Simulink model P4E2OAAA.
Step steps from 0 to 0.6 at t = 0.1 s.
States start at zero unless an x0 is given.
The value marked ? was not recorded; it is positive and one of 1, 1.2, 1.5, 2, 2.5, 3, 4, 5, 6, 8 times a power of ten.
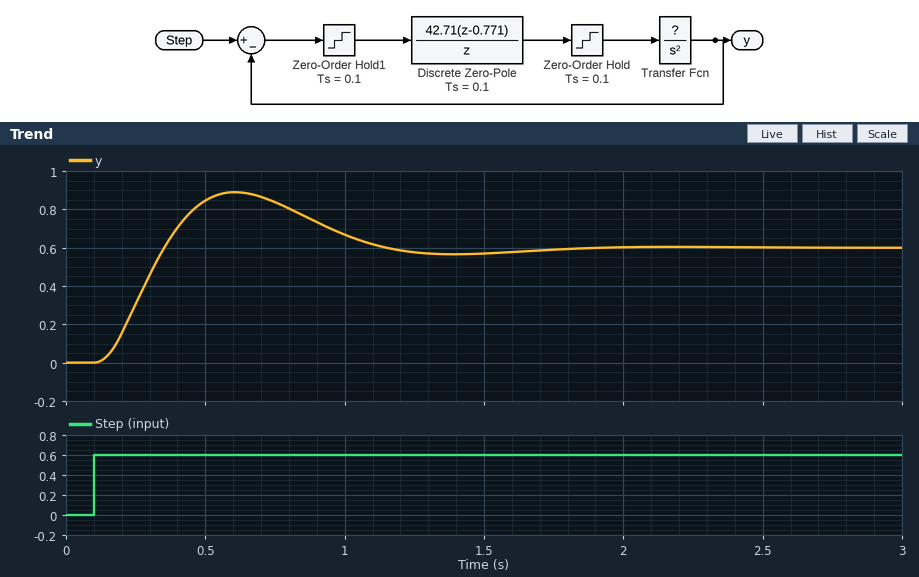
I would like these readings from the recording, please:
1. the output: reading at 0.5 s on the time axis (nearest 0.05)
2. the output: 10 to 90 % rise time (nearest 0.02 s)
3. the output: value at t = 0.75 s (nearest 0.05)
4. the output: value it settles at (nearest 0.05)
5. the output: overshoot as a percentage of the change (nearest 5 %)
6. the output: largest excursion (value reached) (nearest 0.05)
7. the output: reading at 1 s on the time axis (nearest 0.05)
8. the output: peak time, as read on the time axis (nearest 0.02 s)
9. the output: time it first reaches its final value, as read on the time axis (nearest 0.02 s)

0.85
0.16 s
0.85
0.60
50 %
0.90
0.65
0.60 s
0.36 s
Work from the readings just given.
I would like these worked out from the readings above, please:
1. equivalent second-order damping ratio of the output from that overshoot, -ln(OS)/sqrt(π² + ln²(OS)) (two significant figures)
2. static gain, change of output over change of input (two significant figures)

0.22
1.0
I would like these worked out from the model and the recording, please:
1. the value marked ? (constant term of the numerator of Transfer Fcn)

1.2
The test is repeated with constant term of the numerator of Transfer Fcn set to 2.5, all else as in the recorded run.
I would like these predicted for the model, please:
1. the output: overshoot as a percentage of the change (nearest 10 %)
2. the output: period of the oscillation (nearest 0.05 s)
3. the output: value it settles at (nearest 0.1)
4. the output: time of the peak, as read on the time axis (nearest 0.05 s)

80 %
0.60 s
0.6
0.40 s
